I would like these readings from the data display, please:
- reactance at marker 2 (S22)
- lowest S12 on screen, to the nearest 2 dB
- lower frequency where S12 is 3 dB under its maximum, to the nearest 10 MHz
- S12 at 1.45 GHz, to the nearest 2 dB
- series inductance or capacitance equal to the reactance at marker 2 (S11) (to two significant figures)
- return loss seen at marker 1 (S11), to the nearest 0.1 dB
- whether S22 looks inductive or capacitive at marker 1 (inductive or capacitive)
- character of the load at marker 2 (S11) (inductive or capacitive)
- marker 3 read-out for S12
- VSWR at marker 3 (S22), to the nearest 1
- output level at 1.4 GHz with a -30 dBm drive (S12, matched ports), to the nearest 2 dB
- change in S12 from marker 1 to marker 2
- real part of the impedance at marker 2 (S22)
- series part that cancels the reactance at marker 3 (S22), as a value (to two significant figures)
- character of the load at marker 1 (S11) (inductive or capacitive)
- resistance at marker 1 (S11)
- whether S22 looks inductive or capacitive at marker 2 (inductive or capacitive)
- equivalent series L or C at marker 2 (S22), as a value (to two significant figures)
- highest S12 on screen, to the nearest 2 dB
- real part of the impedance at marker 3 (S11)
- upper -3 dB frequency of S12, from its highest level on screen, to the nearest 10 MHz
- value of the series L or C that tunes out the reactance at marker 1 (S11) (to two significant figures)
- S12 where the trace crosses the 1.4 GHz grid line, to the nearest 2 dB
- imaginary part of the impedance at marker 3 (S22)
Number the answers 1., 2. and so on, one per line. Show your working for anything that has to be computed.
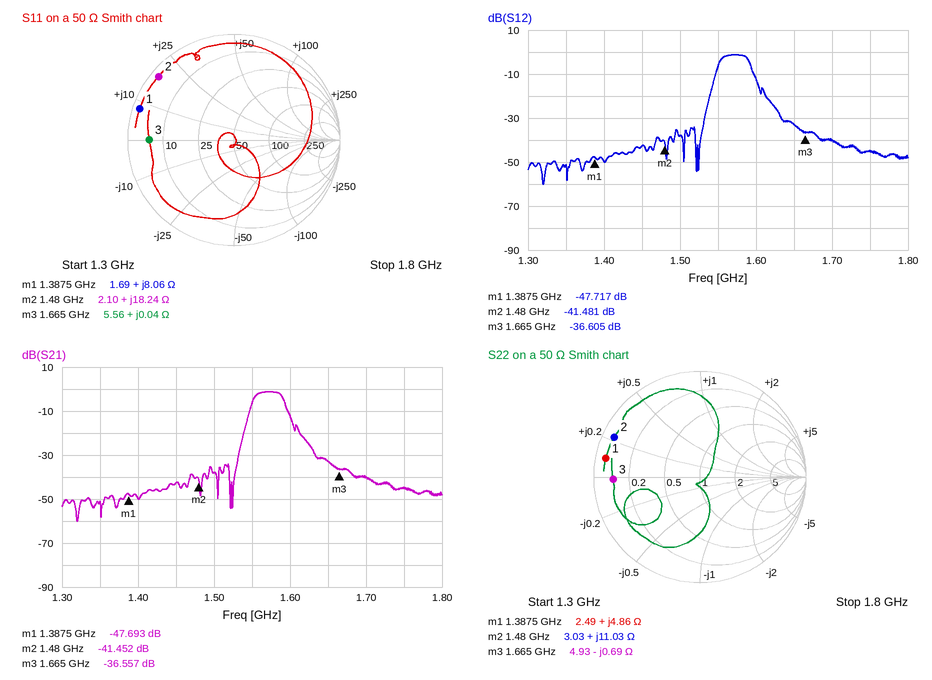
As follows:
1. +11.03 Ω
2. -60 dB
3. 1.55 GHz
4. -42 dB
5. L = 18.24 Ω/(2π × 1.48 GHz) ≈ 2.0 nH
6. 0.6 dB
7. inductive
8. inductive
9. -36.605 dB
10. 10
11. -30 dBm + (-50 dB) = -80 dBm
12. -41.481 − (-47.717) = 6.236 dB
13. 3.03 Ω
14. L = 0.69 Ω/(2π × 1.665 GHz) ≈ 66 pH
15. inductive
16. 1.69 Ω
17. inductive
18. L = 11.03 Ω/(2π × 1.48 GHz) ≈ 1.2 nH
19. -2 dB
20. 5.56 Ω
21. 1.59 GHz
22. C = 1/(2π × 1.3875 GHz × 8.06 Ω) ≈ 14 pF
23. -50 dB
24. -0.69 Ω
